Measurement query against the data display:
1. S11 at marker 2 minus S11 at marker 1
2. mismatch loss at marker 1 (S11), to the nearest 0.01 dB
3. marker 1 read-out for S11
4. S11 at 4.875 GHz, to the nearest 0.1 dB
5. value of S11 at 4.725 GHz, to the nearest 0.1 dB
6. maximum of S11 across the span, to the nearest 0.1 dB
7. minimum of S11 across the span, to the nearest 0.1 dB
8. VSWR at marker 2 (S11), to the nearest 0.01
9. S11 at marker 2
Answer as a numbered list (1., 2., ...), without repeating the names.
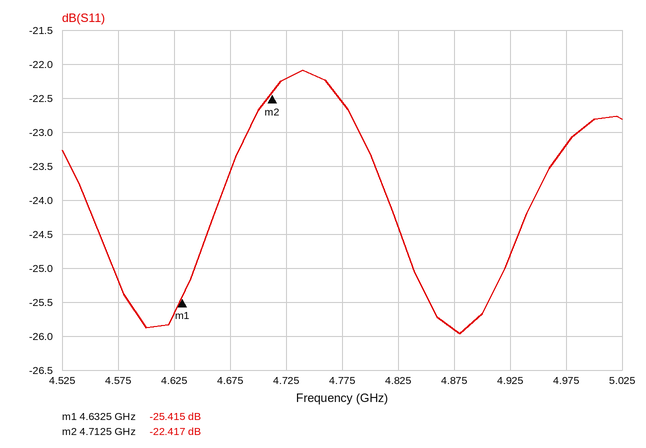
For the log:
1. 2.998 dB
2. 0.01 dB
3. -25.415 dB
4. -25.9 dB
5. -22.2 dB
6. -22.1 dB
7. -26.0 dB
8. 1.16
9. -22.417 dB
